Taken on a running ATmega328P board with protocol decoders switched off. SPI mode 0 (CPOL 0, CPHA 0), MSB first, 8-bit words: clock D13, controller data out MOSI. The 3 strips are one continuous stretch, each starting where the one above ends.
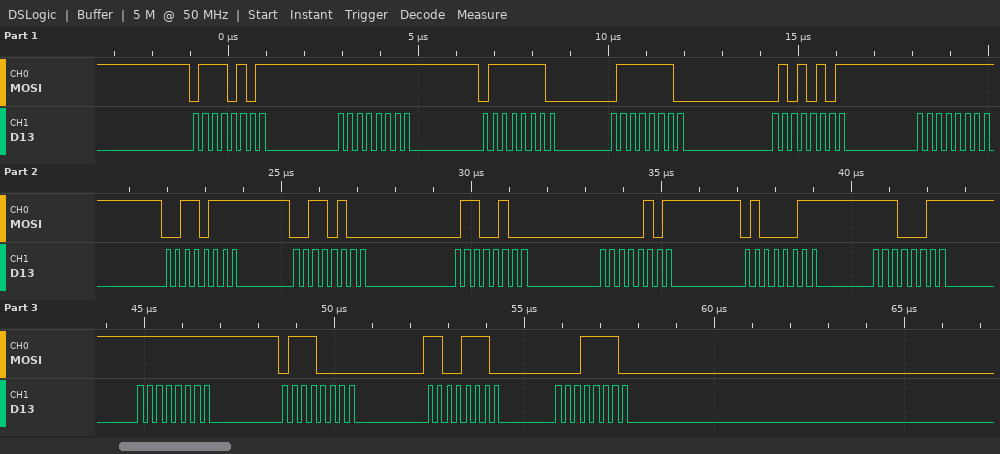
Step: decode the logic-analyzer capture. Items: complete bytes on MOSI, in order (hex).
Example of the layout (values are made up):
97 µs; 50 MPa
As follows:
75 FF 7E 7E 55 FF 37 34 64 05 43 E3 FF 70 CE 1E
